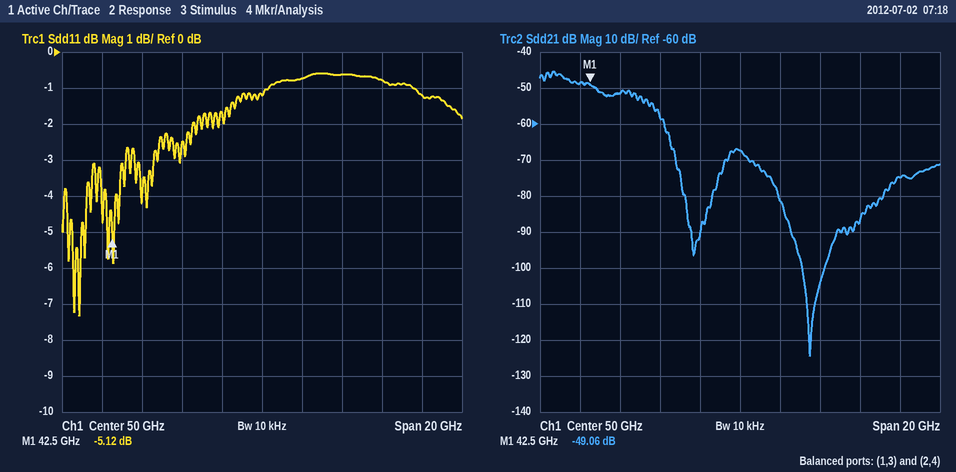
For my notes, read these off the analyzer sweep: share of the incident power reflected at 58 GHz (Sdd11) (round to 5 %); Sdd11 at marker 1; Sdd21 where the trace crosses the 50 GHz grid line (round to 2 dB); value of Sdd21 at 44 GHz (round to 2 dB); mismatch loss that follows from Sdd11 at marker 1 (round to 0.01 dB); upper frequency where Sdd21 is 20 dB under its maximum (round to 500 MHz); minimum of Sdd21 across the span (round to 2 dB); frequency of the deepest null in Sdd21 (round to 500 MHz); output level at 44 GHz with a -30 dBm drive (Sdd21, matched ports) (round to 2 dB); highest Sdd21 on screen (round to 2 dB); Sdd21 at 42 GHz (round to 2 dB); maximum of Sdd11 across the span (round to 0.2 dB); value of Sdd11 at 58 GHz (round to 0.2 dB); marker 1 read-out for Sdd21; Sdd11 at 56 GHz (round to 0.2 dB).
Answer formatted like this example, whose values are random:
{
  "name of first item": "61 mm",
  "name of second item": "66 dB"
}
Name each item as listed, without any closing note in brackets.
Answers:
{
  "share of the incident power reflected at 58 GHz (Sdd11)": "75 %",
  "Sdd11 at marker 1": "-5.12 dB",
  "Sdd21 where the trace crosses the 50 GHz grid line": "-68 dB",
  "value of Sdd21 at 44 GHz": "-52 dB",
  "mismatch loss that follows from Sdd11 at marker 1": "1.60 dB",
  "upper frequency where Sdd21 is 20 dB under its maximum": "46.5 GHz",
  "minimum of Sdd21 across the span": "-124 dB",
  "frequency of the deepest null in Sdd21": "53.5 GHz",
  "output level at 44 GHz with a -30 dBm drive (Sdd21, matched ports)": "-82 dBm",
  "highest Sdd21 on screen": "-46 dB",
  "Sdd21 at 42 GHz": "-48 dB",
  "maximum of Sdd11 across the span": "-0.6 dB",
  "value of Sdd11 at 58 GHz": "-1.2 dB",
  "marker 1 read-out for Sdd21": "-49.06 dB",
  "Sdd11 at 56 GHz": "-0.8 dB"
}
